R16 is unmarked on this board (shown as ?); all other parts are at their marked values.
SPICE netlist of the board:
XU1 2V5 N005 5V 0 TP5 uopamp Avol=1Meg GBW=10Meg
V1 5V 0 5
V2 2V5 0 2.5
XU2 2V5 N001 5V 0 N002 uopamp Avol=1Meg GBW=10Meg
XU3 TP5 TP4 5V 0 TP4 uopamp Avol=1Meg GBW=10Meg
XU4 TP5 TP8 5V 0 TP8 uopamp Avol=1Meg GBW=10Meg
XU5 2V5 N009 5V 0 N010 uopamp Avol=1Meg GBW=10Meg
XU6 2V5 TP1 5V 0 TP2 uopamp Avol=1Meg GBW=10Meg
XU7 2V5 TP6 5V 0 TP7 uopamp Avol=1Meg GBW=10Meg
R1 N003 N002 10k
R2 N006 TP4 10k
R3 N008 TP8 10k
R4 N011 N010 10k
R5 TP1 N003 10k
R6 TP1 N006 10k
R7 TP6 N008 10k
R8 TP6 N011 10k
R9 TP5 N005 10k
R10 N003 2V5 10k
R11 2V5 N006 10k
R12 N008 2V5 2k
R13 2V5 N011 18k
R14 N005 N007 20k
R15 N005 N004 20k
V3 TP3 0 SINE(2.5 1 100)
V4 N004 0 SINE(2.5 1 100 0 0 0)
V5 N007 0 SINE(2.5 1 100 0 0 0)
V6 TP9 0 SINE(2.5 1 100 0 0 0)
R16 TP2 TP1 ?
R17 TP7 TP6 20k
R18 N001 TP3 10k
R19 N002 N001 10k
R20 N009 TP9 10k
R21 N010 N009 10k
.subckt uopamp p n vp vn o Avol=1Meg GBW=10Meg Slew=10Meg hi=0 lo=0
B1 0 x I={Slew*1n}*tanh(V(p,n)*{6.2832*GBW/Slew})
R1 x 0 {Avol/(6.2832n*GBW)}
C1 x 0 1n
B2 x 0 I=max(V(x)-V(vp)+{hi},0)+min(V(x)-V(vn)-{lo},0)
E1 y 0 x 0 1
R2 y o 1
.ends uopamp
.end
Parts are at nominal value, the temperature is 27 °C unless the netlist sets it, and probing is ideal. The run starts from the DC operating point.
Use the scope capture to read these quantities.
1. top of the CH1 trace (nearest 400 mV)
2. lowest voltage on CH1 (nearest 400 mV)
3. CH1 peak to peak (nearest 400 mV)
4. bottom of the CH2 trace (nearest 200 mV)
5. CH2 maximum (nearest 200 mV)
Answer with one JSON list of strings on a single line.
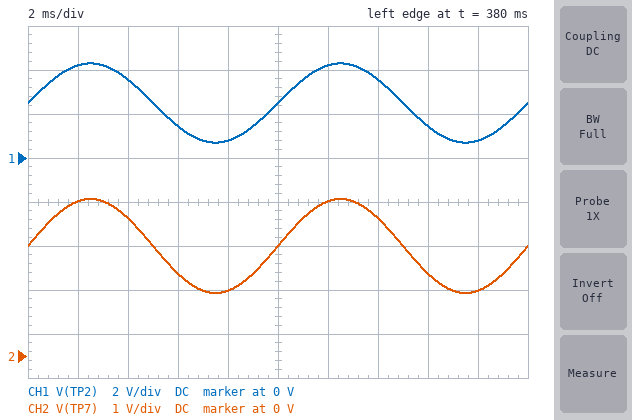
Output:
["4.4 V", "800 mV", "3.6 V", "1.4 V", "3.6 V"]
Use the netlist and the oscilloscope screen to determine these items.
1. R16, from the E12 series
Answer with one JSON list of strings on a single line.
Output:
["27 kΩ"]
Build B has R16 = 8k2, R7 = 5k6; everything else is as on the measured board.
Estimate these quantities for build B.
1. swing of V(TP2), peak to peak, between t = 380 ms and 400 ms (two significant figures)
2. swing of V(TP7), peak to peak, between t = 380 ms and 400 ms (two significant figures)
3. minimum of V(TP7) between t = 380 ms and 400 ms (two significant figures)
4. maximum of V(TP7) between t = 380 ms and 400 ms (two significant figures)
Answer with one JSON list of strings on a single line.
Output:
["1.1 V", "2.5 V", "1.3 V", "3.7 V"]
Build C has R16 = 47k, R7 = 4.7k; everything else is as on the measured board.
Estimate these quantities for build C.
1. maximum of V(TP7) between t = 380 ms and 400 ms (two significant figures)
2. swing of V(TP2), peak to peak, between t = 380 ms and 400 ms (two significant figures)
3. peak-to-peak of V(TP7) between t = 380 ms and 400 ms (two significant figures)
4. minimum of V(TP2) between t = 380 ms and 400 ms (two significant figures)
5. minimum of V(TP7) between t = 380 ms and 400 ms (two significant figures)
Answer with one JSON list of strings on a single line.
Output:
["3.8 V", "5.0 V", "2.6 V", "-4.9 mV", "1.2 V"]
